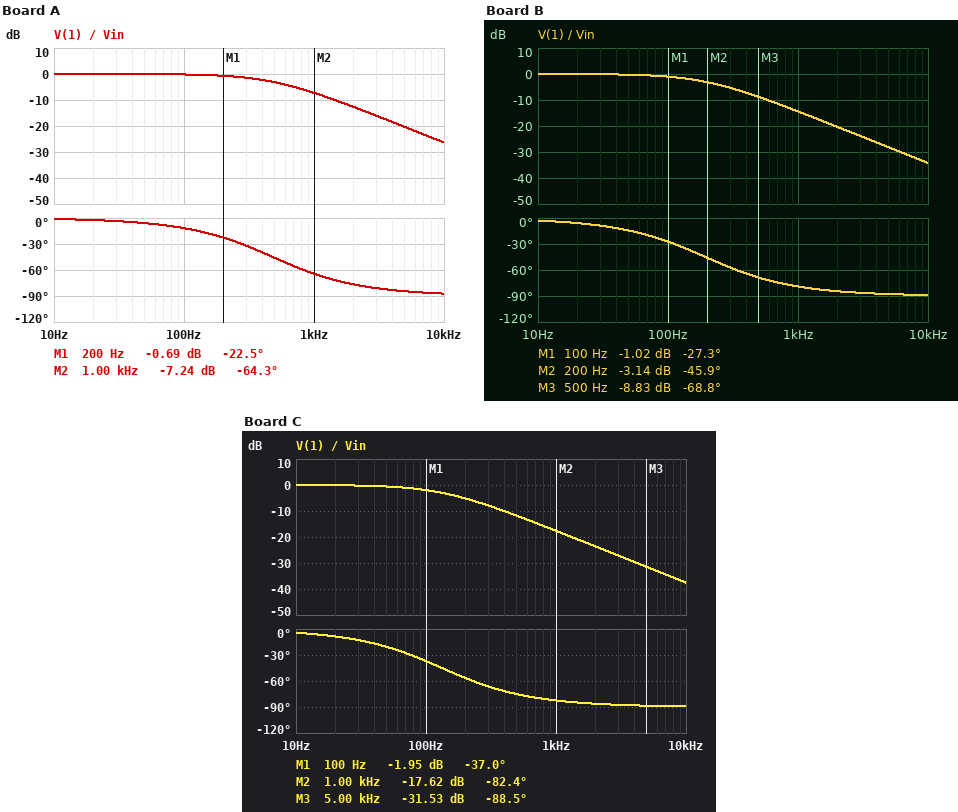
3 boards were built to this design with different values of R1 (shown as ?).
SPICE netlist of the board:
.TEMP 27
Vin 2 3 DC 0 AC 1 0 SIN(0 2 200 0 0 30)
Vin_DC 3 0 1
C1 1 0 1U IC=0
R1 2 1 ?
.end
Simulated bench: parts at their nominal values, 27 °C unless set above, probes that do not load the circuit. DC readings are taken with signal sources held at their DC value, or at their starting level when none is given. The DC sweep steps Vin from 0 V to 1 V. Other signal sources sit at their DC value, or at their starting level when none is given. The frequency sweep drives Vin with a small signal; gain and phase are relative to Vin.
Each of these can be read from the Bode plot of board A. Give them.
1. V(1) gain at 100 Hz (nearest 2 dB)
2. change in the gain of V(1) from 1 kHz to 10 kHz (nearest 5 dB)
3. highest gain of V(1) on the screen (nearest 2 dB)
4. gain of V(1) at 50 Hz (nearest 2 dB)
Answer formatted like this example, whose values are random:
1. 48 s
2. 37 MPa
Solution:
1. 0 dB
2. -20 dB
3. 0 dB
4. 0 dB
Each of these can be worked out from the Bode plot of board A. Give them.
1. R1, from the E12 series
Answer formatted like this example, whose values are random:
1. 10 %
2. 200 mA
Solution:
1. 330 Ω
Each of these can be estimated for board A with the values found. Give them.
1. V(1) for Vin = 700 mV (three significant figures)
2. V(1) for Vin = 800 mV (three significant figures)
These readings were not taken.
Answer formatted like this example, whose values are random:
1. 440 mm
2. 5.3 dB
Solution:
1. 1.70 V
2. 1.80 V
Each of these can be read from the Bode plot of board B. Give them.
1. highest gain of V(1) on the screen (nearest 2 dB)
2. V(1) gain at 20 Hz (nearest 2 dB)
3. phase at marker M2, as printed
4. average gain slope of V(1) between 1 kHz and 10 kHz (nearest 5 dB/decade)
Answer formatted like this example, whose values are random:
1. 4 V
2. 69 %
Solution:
1. 0 dB
2. 0 dB
3. -45.9 deg
4. -20 dB/decade
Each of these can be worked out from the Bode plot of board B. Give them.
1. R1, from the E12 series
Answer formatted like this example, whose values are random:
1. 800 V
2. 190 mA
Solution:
1. 820 Ω
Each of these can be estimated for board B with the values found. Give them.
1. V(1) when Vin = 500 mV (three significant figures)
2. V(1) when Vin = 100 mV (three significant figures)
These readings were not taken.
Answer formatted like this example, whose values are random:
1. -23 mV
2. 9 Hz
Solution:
1. 1.50 V
2. 1.10 V
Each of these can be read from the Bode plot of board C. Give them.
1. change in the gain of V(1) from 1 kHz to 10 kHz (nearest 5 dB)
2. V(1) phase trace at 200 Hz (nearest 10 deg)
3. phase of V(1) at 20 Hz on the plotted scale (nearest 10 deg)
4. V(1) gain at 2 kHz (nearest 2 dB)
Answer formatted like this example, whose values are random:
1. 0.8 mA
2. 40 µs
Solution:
1. -20 dB
2. -60 deg
3. -10 deg
4. -24 dB
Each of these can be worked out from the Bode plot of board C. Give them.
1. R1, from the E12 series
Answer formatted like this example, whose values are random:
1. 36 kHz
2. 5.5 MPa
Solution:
1. 1.2 kΩ
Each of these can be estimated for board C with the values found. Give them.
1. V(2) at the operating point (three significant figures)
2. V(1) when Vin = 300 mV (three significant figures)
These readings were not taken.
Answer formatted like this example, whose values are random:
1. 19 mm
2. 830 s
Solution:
1. 1.00 V
2. 1.30 V
